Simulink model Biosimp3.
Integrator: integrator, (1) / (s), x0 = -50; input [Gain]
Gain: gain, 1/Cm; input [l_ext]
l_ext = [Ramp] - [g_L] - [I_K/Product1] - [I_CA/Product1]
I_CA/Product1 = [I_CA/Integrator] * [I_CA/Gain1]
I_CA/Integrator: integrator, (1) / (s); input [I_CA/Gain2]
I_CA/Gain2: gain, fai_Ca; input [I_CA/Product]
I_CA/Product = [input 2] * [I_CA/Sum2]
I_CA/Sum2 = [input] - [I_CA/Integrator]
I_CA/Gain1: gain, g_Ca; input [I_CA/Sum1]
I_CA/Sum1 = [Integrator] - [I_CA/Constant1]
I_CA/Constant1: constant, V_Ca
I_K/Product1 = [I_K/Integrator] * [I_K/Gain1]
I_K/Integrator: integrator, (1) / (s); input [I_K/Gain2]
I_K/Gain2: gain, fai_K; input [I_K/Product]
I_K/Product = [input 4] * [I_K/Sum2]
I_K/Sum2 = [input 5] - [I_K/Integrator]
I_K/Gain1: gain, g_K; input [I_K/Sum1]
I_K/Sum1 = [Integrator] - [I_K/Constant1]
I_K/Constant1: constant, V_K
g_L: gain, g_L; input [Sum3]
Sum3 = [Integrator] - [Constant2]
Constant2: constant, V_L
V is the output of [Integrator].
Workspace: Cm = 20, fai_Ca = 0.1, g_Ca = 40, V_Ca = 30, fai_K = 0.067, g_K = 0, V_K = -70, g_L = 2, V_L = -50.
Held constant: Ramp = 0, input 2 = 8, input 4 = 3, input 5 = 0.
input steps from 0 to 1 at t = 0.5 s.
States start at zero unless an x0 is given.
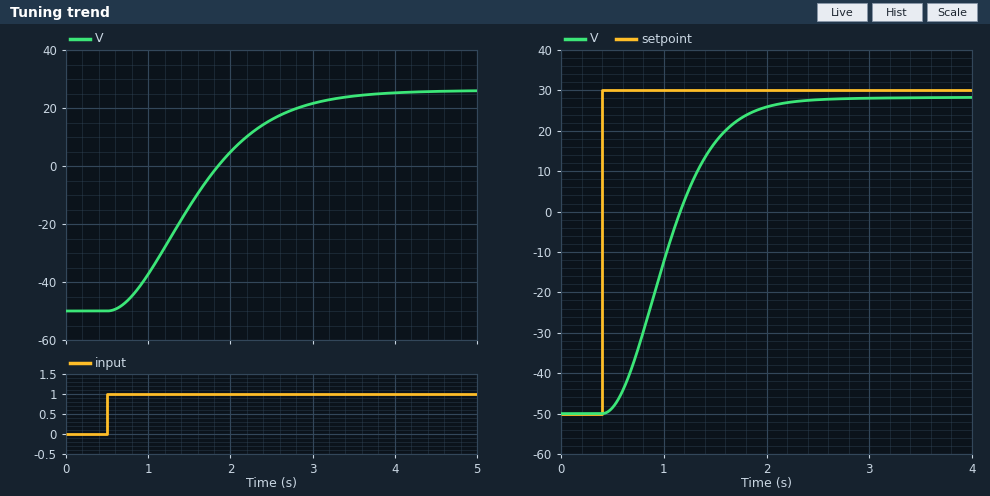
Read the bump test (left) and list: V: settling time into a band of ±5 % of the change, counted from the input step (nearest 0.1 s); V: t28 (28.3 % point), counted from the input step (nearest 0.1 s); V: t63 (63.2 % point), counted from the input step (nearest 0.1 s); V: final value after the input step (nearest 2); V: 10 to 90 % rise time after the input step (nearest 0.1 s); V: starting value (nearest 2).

2.6 s
0.7 s
1.3 s
26
1.8 s
-50
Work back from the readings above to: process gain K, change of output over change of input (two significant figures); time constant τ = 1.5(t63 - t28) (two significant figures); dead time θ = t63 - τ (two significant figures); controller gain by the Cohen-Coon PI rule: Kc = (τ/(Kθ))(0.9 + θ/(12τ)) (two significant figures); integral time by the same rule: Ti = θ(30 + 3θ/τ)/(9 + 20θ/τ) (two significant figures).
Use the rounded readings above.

76
0.90 s
0.40 s
0.028
0.70 s
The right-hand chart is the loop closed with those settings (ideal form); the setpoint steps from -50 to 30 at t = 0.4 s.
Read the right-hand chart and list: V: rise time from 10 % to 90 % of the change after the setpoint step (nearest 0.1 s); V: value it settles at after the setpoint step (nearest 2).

1.0 s
28
